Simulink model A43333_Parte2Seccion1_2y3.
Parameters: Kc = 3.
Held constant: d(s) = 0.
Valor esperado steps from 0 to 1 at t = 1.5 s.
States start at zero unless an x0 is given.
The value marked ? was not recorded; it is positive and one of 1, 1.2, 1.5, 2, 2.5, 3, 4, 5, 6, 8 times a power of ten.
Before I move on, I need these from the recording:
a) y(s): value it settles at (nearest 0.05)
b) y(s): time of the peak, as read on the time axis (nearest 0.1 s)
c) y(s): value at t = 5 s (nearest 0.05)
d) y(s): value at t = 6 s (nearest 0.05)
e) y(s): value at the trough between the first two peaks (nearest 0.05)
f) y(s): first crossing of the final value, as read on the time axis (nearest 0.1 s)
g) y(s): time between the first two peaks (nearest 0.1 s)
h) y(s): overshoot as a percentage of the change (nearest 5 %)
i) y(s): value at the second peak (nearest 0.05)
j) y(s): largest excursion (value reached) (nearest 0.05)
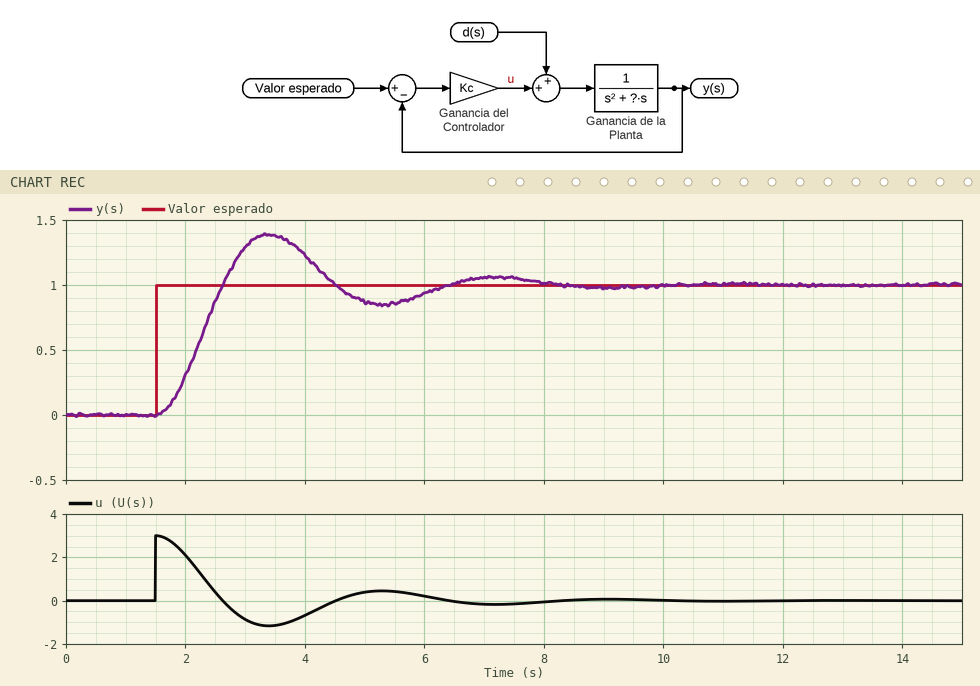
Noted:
1.00
3.4 s
0.85
0.95
0.85
2.6 s
3.8 s
40 %
1.05
1.40
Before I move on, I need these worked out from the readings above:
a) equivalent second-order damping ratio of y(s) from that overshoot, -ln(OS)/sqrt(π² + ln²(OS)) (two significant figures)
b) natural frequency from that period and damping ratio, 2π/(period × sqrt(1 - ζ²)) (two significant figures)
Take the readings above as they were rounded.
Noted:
0.28
1.7 rad/s
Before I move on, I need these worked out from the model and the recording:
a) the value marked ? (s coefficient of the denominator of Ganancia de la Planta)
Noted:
1
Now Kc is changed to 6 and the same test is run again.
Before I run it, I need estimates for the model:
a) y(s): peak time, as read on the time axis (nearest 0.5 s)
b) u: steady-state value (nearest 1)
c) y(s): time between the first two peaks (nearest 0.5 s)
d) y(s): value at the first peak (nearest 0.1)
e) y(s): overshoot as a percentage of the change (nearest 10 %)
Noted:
3.0 s
0
2.5 s
1.5
50 %
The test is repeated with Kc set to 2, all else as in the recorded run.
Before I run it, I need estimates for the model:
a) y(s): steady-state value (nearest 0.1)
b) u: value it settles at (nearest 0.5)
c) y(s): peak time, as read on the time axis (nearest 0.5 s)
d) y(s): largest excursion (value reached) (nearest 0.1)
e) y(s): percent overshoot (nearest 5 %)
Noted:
1.0
0.0
4.0 s
1.3
30 %
